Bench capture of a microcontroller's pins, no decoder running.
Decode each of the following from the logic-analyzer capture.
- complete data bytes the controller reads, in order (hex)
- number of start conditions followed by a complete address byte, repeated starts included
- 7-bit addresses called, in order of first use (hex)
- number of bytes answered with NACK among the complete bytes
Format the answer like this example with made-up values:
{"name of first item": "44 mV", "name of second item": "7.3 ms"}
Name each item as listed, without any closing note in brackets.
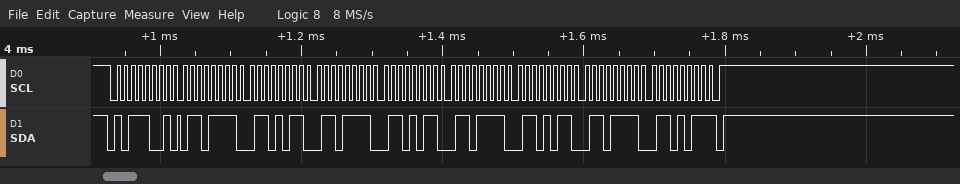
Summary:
{"complete data bytes the controller reads, in order": "6F 6B 6F 6B 6F 6B 6F 6B", "number of start conditions followed by a complete address byte, repeated starts included": "1", "7-bit addresses called, in order of first use": "0x5C", "number of bytes answered with NACK among the complete bytes": "1"}
